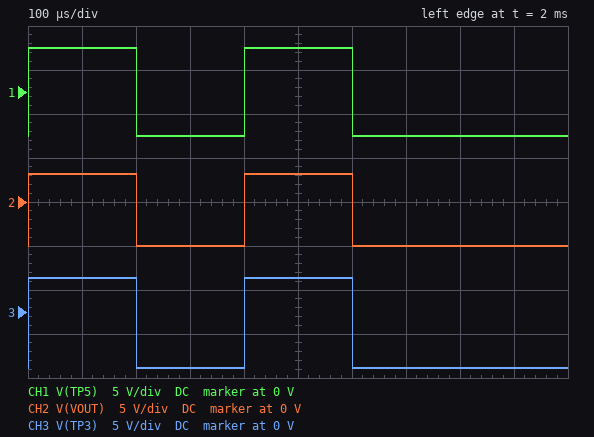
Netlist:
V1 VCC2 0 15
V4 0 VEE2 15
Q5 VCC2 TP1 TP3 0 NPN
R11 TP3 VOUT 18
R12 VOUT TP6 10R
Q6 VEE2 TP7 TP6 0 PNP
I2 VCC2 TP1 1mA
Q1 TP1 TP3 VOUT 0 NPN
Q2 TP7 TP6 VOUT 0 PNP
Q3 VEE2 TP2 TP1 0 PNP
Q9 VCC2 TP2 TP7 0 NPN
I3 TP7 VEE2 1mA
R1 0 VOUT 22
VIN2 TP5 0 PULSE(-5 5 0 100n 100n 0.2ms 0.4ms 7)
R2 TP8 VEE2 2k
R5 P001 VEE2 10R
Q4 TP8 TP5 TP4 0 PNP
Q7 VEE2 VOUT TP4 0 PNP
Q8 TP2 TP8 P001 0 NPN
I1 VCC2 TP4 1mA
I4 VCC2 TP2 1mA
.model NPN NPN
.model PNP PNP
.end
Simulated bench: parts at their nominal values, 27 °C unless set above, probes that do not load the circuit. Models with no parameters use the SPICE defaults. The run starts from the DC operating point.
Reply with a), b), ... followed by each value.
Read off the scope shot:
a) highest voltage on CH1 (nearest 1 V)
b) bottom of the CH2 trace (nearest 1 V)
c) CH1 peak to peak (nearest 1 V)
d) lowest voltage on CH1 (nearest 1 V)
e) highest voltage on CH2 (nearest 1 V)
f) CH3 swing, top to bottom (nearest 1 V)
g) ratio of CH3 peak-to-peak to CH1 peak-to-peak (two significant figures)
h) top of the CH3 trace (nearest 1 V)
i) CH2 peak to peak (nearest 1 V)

a) 5 V
b) -5 V
c) 10 V
d) -5 V
e) 3 V
f) 10 V
g) 1.0
h) 4 V
i) 8 V
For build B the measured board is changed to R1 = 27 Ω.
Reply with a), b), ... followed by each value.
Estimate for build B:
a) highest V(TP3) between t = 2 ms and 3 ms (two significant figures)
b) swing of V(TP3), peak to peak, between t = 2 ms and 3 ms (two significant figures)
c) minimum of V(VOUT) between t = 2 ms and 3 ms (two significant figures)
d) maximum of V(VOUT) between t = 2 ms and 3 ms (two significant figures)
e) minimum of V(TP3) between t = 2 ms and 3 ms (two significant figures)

a) 4.6 V
b) 11 V
c) -5.0 V
d) 3.9 V
e) -6.0 V
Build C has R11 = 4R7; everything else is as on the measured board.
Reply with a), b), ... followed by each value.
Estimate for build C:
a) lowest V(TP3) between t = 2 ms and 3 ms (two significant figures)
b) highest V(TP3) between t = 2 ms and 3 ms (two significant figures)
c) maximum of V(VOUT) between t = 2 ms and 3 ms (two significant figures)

a) -5.4 V
b) 4.9 V
c) 4.4 V
